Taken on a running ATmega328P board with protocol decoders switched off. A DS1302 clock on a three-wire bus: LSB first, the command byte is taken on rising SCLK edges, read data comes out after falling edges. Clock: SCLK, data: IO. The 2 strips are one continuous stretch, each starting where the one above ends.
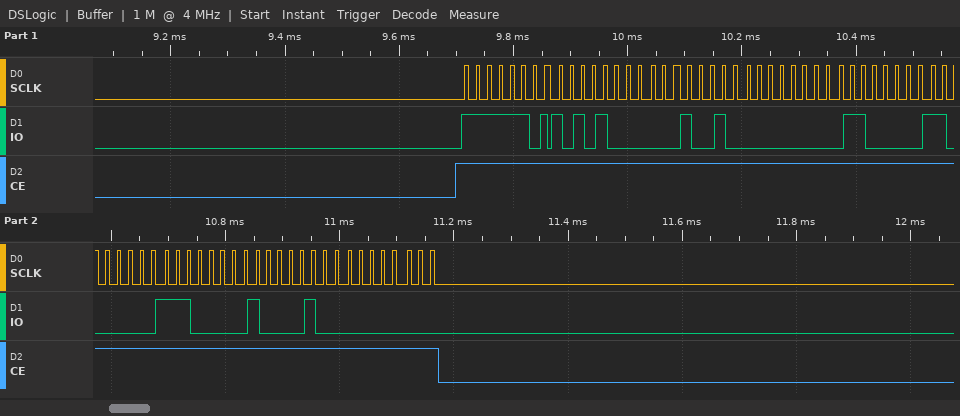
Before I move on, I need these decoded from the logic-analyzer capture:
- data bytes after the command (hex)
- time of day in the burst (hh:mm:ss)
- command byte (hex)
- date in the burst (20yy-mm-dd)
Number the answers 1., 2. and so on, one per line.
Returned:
1. 15 48 00 06 03 07 21 00
2. 00:48:15
3. 0xBF
4. 2021-03-06
